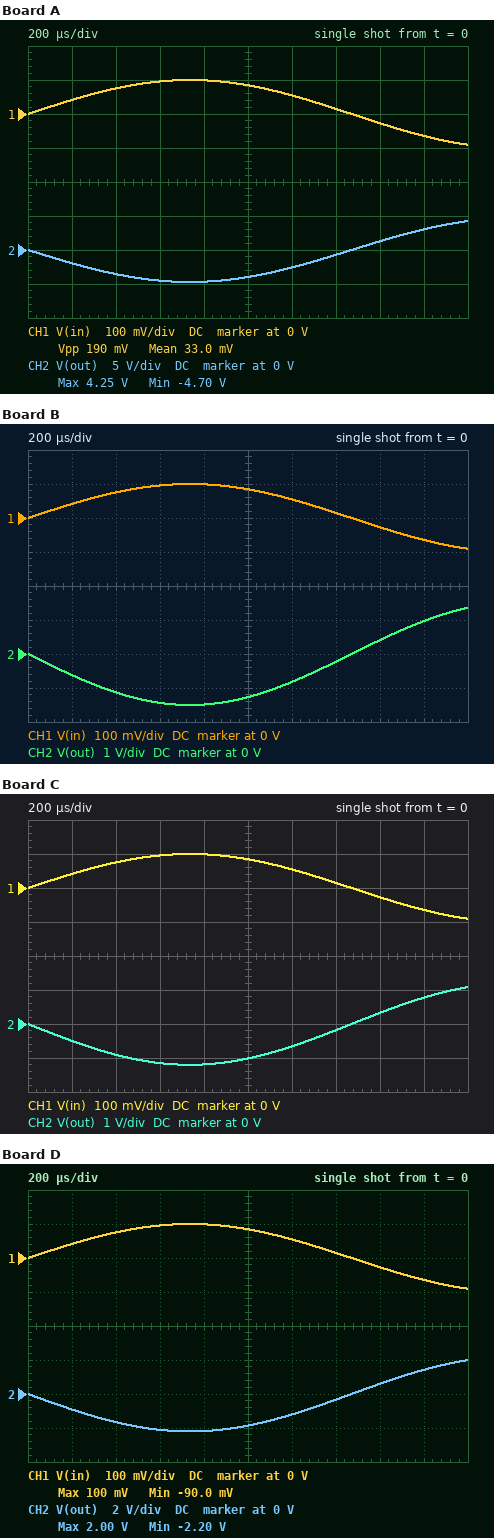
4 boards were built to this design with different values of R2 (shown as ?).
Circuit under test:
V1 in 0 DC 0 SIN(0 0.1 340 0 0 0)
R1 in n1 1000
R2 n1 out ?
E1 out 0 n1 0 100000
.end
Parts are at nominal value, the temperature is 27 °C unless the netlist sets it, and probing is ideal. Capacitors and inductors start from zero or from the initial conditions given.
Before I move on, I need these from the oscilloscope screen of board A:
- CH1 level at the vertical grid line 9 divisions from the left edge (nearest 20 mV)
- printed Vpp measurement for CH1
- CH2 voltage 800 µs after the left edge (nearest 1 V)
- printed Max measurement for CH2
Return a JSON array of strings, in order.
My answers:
["-60 mV", "190 mV", "-5 V", "4.25 V"]
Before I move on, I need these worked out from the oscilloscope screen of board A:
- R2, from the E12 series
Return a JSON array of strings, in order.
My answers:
["47 kΩ"]
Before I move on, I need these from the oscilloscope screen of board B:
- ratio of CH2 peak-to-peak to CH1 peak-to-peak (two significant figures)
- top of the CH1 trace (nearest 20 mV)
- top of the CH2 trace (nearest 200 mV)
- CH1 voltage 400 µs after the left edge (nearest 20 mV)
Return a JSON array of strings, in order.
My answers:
["15", "100 mV", "1.4 V", "80 mV"]
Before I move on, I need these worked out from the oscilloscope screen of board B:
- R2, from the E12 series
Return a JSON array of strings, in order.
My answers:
["15 kΩ"]
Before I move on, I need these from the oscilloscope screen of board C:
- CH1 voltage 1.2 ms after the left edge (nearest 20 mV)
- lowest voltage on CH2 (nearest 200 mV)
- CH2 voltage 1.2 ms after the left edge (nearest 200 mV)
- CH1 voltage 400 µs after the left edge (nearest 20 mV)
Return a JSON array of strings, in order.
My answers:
["60 mV", "-1.2 V", "-600 mV", "80 mV"]
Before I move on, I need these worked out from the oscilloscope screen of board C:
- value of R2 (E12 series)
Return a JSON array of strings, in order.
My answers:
["12 kΩ"]
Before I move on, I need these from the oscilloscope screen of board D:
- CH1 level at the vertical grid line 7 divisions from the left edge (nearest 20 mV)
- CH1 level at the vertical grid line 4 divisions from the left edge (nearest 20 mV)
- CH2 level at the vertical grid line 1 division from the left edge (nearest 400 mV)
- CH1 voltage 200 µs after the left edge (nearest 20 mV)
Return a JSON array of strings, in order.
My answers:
["20 mV", "100 mV", "-800 mV", "40 mV"]
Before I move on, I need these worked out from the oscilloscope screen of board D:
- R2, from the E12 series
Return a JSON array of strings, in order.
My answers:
["22 kΩ"]
